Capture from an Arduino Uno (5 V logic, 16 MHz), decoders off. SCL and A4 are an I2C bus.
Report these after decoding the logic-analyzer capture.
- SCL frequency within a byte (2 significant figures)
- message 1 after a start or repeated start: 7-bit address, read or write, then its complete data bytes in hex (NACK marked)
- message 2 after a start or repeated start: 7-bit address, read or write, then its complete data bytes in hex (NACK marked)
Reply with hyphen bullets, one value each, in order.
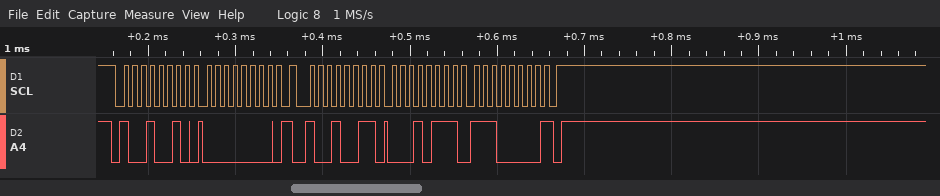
- 100 kHz
- 0x49 write: 00
- 0x49 read: 17 E0 NACK
